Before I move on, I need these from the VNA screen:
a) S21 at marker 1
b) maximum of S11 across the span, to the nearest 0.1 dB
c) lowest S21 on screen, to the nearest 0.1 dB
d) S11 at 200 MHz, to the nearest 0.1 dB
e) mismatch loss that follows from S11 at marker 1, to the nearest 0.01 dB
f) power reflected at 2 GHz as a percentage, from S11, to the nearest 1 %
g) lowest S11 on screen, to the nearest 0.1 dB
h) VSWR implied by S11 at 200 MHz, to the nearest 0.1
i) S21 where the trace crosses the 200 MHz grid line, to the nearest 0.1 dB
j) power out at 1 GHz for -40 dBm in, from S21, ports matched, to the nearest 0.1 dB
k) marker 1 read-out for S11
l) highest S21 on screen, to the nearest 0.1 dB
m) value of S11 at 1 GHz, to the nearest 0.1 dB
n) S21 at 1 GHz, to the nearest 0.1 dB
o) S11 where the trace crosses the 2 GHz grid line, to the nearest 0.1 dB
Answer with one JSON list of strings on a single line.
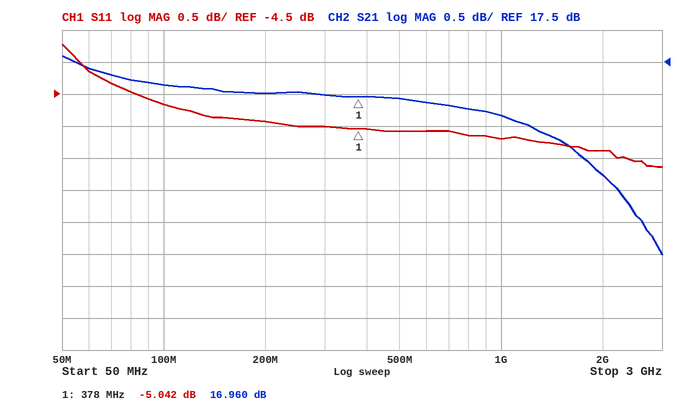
["16.960 dB", "-3.7 dB", "14.5 dB", "-4.9 dB", "1.63 dB", "29 %", "-5.6 dB", "3.6", "17.0 dB", "-23.3 dBm", "-5.042 dB", "17.6 dB", "-5.2 dB", "16.7 dB", "-5.4 dB"]
